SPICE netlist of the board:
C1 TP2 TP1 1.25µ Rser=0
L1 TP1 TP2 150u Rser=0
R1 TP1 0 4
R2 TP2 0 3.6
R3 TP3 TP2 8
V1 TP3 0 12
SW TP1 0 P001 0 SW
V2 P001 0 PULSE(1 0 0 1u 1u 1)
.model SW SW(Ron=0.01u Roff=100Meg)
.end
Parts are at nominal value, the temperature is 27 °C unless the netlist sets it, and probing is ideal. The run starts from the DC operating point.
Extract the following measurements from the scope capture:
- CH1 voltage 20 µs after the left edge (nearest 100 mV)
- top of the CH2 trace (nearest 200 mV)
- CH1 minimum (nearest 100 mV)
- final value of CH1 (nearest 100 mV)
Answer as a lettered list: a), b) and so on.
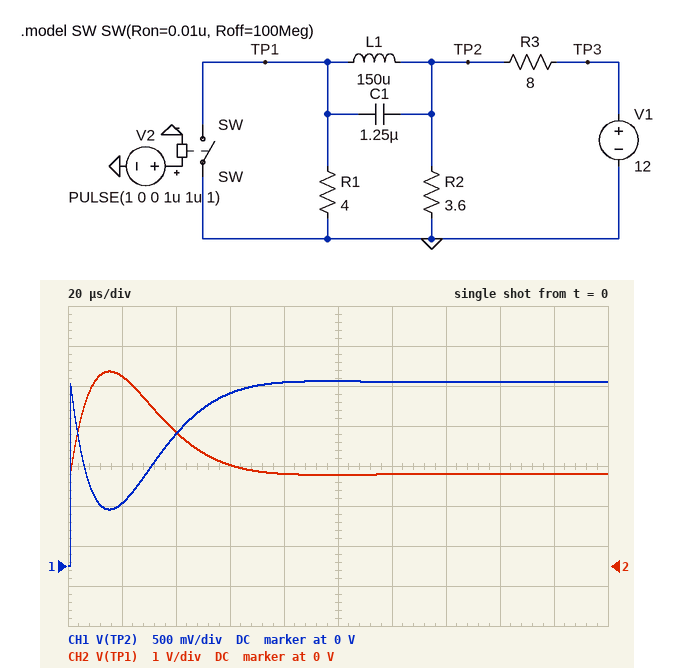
a) 800 mV
b) 4.8 V
c) 0 V
d) 2.3 V
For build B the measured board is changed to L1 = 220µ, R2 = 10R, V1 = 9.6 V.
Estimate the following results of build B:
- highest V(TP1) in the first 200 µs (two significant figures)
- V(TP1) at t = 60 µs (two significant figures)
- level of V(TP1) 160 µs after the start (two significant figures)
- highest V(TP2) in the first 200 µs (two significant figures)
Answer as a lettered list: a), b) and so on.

a) 4.1 V
b) 2.8 V
c) 2.5 V
d) 2.6 V
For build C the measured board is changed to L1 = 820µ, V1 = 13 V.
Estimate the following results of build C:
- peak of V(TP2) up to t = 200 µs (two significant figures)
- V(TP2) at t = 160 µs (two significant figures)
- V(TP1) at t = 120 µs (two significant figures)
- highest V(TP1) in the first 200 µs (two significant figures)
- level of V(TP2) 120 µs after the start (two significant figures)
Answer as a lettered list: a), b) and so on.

a) 2.5 V
b) 1.7 V
c) 4.2 V
d) 6.0 V
e) 1.4 V
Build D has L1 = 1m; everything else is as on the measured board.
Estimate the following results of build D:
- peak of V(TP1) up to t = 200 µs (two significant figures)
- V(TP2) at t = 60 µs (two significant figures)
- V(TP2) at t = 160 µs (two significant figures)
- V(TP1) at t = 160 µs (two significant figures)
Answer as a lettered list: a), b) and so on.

a) 5.6 V
b) 580 mV
c) 1.4 V
d) 3.7 V
